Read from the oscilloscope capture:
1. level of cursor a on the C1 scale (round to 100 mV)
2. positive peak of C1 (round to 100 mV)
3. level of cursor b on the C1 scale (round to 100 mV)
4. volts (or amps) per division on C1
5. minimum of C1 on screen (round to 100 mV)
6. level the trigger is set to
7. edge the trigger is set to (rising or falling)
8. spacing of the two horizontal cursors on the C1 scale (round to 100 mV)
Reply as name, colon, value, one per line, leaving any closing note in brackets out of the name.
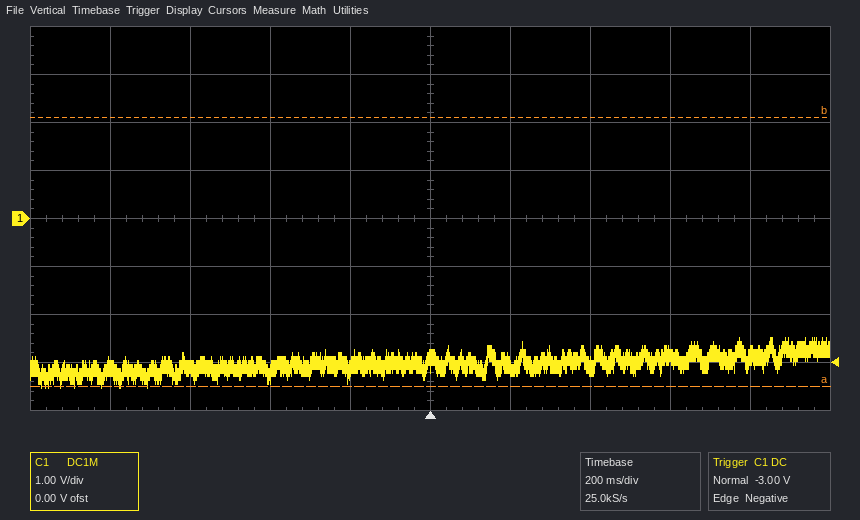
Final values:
level of cursor a on the C1 scale: -3.5 V
positive peak of C1: -2.5 V
level of cursor b on the C1 scale: 2.1 V
volts (or amps) per division on C1: 1 V
minimum of C1 on screen: -3.5 V
level the trigger is set to: -3.00 V
edge the trigger is set to: falling
spacing of the two horizontal cursors on the C1 scale: 5.6 V
